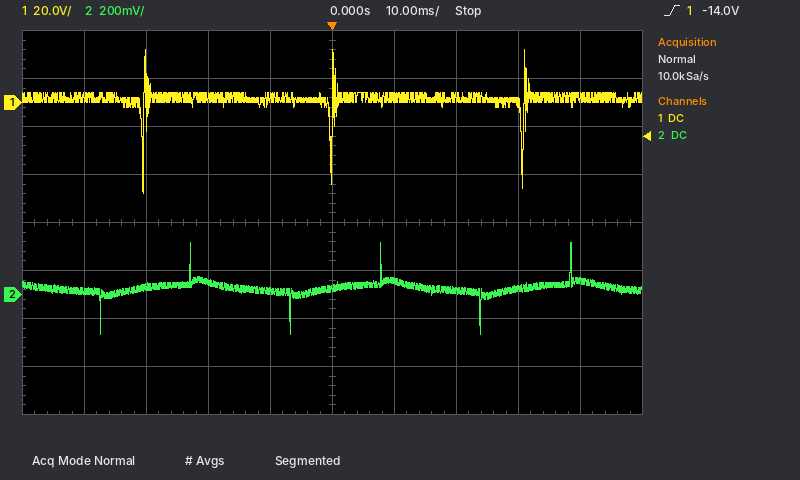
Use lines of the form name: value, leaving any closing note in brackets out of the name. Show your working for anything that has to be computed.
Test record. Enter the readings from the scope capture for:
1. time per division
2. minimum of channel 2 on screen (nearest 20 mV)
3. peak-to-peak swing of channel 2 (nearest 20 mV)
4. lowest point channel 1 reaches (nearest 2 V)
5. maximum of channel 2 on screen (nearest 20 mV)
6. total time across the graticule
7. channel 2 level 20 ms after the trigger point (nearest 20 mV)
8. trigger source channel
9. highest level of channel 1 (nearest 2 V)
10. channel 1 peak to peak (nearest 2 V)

time per division: 10 ms
minimum of channel 2 on screen: -160 mV
peak-to-peak swing of channel 2: 220 mV − (-160 mV) = 380 mV
lowest point channel 1 reaches: -38 V
maximum of channel 2 on screen: 220 mV
total time across the graticule: 100 ms
channel 2 level 20 ms after the trigger point: 20 mV
trigger source channel: channel 1
highest level of channel 1: 22 V
channel 1 peak to peak: 22 V − (-38 V) = 60 V
